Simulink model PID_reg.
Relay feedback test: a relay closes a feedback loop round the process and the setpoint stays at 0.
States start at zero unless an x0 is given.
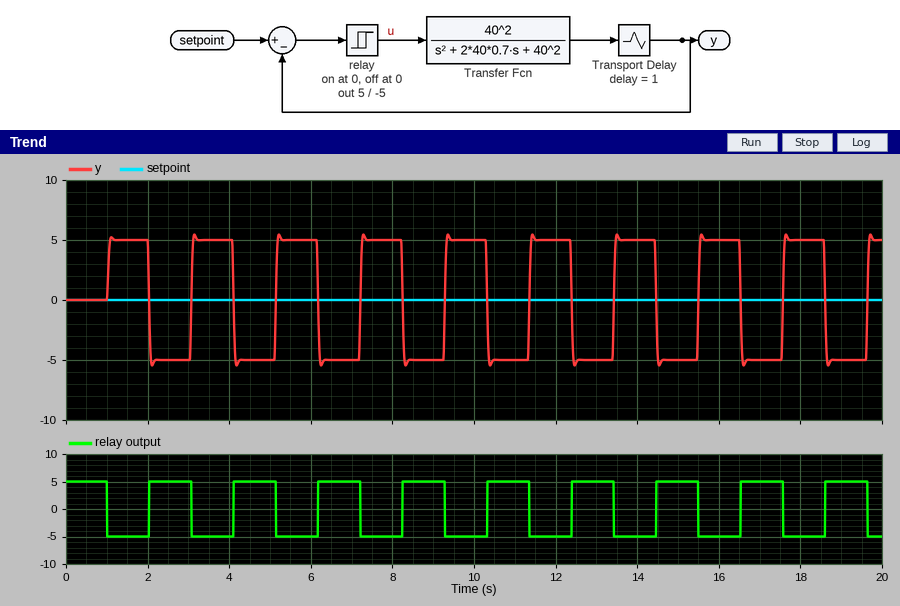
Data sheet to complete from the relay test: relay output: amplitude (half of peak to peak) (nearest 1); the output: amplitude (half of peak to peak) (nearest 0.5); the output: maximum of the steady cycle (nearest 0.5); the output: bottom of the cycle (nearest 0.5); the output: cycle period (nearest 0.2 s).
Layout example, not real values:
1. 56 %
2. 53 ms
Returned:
1. 5
2. 5.5
3. 5.5
4. -5.5
5. 2.0 s
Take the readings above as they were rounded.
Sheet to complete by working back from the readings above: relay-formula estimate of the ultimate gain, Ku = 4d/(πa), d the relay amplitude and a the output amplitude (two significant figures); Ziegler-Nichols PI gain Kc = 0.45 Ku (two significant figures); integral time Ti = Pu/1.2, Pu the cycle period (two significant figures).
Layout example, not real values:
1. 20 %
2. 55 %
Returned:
1. 1.2
2. 0.54
3. 1.7 s
